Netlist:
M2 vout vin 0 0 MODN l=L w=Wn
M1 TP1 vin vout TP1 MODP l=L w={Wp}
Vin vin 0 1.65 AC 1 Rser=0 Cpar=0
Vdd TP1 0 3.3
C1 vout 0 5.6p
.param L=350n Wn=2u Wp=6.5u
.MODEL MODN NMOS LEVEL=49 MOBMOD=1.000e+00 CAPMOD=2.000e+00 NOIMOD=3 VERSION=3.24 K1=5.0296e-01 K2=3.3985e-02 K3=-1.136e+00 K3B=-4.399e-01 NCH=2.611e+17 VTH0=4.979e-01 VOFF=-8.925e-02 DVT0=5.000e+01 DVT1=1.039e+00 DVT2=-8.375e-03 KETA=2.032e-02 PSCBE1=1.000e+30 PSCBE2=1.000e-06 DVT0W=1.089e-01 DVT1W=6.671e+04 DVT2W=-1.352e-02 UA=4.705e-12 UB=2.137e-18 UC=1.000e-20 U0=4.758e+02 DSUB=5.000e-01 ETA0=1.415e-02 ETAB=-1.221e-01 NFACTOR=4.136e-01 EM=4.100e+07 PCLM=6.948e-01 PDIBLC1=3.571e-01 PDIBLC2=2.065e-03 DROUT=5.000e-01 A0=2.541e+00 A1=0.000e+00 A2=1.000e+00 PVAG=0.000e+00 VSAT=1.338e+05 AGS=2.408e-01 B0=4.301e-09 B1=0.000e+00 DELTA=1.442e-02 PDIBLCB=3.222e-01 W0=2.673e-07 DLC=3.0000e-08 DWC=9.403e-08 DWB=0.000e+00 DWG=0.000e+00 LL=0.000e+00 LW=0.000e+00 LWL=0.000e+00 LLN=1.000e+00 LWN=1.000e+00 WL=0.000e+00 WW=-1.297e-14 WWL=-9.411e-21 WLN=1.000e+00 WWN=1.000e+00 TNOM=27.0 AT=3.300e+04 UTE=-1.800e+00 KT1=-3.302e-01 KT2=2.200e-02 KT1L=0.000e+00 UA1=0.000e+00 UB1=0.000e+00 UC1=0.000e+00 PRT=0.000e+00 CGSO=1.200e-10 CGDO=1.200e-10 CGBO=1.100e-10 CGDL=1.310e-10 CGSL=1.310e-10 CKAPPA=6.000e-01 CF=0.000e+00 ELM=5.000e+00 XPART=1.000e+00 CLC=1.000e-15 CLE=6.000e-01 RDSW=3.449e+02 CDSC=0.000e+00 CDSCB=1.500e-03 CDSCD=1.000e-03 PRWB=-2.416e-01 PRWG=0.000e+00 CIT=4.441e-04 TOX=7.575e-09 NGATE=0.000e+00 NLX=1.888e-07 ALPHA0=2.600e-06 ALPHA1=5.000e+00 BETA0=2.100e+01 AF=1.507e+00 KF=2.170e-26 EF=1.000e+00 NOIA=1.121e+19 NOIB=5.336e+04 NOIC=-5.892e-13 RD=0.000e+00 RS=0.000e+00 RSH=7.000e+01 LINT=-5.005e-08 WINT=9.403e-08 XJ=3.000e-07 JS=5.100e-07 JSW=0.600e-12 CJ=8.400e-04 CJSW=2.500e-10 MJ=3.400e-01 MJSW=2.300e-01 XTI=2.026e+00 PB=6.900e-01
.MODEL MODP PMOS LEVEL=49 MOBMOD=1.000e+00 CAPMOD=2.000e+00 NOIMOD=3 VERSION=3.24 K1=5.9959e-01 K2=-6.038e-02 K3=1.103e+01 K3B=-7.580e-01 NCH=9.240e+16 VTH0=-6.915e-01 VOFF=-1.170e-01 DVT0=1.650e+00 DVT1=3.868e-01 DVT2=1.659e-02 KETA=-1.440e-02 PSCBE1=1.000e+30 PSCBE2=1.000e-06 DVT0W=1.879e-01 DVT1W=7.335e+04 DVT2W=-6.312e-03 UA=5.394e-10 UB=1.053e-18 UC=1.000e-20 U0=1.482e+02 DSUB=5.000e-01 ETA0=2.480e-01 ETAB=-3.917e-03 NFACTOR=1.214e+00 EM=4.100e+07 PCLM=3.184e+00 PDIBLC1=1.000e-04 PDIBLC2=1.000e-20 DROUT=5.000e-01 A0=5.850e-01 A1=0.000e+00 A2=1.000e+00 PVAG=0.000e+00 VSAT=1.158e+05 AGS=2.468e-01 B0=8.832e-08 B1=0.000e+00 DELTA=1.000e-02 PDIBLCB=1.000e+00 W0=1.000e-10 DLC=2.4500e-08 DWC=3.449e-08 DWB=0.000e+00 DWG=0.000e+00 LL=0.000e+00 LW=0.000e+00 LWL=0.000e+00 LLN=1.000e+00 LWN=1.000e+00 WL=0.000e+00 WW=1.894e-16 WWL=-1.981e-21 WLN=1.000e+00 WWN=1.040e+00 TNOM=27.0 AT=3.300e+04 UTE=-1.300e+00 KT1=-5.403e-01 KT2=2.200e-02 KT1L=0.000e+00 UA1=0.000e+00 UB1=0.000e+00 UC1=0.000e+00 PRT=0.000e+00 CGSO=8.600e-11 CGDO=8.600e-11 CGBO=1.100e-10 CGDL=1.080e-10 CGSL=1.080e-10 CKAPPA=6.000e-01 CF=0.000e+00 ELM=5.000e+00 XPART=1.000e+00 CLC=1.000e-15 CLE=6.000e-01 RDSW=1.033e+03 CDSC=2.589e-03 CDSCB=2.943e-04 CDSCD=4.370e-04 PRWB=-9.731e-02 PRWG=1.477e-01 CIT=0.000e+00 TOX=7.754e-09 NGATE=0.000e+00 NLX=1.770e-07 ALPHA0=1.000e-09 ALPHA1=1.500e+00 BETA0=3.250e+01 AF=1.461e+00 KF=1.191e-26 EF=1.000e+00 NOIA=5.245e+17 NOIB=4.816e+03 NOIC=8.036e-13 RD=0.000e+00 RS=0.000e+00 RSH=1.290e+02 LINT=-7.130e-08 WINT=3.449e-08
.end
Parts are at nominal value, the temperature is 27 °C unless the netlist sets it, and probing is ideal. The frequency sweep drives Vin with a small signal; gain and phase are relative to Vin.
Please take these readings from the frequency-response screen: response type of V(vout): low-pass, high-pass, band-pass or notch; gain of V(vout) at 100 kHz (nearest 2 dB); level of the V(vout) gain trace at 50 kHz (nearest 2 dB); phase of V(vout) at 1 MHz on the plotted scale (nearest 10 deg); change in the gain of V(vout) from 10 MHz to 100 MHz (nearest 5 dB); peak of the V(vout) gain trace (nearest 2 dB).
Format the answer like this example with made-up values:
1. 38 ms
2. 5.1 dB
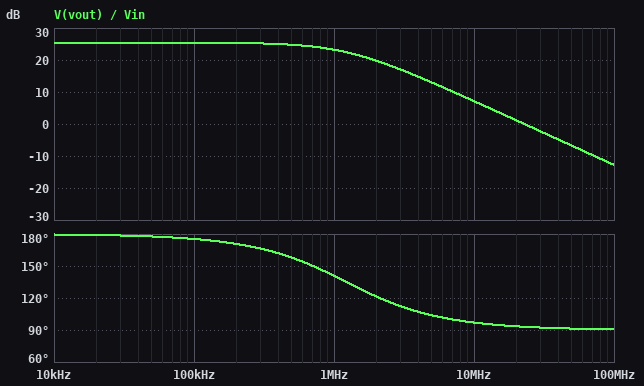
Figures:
1. low-pass
2. 26 dB
3. 26 dB
4. 140 deg
5. -20 dB
6. 26 dB
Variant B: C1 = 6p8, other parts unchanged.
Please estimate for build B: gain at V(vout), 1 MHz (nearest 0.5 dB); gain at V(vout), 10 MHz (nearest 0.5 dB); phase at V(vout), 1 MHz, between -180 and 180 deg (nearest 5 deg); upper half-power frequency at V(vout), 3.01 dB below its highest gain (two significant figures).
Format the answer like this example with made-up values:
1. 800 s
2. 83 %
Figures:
1. 22.5 dB
2. 5.5 dB
3. 135 deg
4. 1.0 MHz
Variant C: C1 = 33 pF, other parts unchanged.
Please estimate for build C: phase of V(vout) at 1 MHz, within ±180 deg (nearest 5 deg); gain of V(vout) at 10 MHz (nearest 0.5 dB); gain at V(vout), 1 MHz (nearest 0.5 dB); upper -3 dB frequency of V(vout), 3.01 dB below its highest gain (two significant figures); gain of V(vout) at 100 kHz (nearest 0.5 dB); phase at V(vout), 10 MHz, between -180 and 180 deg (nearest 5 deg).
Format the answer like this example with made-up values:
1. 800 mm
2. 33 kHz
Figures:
1. 100 deg
2. -8.0 dB
3. 11.5 dB
4. 210 kHz
5. 24.5 dB
6. 90 deg
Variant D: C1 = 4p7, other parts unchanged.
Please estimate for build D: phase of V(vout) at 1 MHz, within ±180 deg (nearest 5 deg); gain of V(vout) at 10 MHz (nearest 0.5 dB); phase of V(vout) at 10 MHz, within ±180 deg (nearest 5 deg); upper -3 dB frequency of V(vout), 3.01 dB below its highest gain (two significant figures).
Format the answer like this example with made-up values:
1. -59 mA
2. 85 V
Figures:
1. 145 deg
2. 8.5 dB
3. 100 deg
4. 1.5 MHz
